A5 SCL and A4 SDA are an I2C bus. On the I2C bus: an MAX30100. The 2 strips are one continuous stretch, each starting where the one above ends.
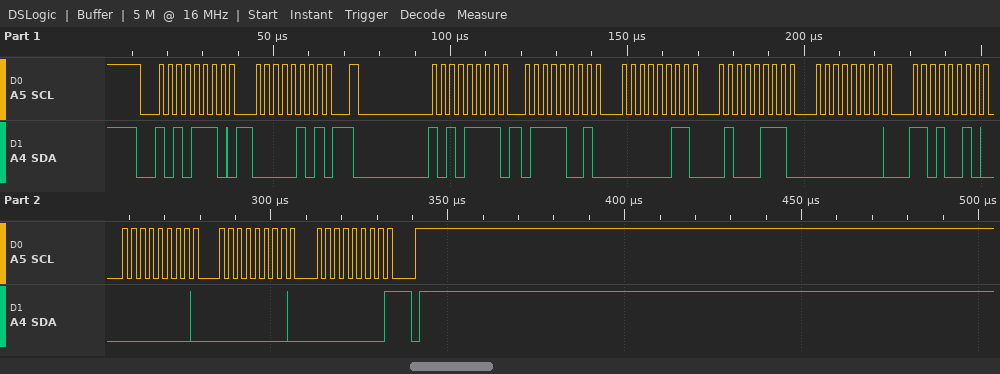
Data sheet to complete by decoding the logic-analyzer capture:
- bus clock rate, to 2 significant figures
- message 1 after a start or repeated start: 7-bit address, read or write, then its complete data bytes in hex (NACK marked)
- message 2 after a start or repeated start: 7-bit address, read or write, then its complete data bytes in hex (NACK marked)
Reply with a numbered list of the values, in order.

1. 400 kHz
2. 0x57 write: 05
3. 0x57 read: 79 03 47 00 D2 00 00 00 NACK
